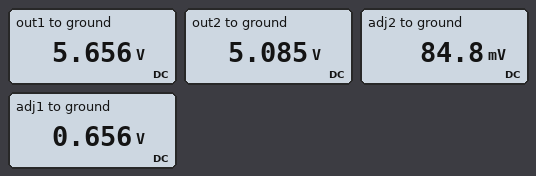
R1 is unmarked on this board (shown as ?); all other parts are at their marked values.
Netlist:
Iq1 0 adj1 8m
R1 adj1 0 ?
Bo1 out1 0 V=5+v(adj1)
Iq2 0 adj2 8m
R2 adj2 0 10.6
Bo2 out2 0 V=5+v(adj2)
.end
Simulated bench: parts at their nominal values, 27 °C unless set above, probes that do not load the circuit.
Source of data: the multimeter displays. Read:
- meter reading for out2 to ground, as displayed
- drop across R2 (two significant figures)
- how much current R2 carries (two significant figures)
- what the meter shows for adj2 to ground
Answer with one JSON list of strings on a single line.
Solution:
["5.085 V", "85 mV", "8.0 mA", "84.8 mV"]
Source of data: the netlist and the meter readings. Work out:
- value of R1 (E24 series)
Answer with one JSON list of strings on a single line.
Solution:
["82 Ω"]
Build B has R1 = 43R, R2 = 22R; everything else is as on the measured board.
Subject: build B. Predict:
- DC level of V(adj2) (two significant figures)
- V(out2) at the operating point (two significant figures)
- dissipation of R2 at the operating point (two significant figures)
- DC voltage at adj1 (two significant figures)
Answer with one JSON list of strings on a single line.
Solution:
["180 mV", "5.2 V", "1.4 mW", "340 mV"]
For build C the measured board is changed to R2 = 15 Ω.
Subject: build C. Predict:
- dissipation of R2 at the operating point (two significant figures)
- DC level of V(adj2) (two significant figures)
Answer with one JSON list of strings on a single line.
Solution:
["960 µW", "120 mV"]
